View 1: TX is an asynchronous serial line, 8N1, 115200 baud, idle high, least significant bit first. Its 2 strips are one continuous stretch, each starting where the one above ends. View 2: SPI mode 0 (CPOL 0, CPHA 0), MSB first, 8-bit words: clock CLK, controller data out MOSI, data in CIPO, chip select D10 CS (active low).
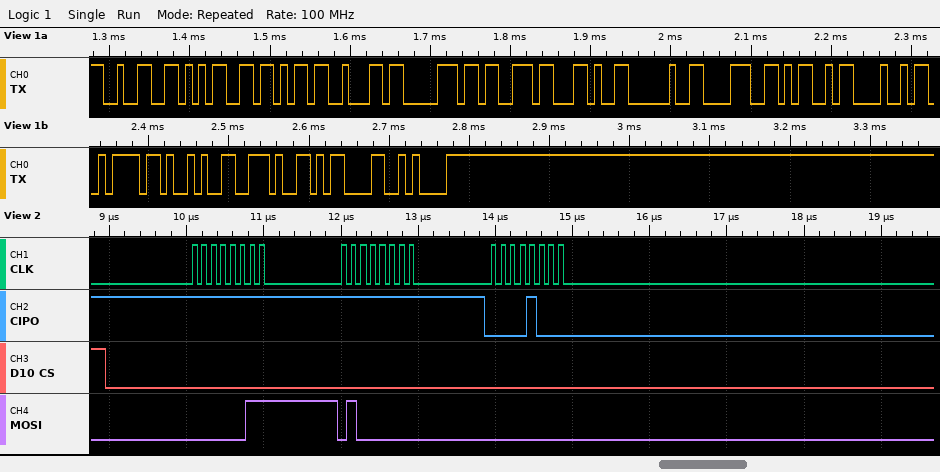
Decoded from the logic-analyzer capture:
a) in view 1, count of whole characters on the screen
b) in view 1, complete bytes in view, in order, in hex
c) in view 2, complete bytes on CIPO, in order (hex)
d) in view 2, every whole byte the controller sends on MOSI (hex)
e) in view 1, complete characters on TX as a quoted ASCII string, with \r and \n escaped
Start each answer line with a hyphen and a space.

- 16
- 32 35 6B 62 70 73 2C 20 38 4D 48 7A 29 2E 0D 0A
- FF FF 08
- 03 40 00
- "25kbps, 8MHz).\r\n"
